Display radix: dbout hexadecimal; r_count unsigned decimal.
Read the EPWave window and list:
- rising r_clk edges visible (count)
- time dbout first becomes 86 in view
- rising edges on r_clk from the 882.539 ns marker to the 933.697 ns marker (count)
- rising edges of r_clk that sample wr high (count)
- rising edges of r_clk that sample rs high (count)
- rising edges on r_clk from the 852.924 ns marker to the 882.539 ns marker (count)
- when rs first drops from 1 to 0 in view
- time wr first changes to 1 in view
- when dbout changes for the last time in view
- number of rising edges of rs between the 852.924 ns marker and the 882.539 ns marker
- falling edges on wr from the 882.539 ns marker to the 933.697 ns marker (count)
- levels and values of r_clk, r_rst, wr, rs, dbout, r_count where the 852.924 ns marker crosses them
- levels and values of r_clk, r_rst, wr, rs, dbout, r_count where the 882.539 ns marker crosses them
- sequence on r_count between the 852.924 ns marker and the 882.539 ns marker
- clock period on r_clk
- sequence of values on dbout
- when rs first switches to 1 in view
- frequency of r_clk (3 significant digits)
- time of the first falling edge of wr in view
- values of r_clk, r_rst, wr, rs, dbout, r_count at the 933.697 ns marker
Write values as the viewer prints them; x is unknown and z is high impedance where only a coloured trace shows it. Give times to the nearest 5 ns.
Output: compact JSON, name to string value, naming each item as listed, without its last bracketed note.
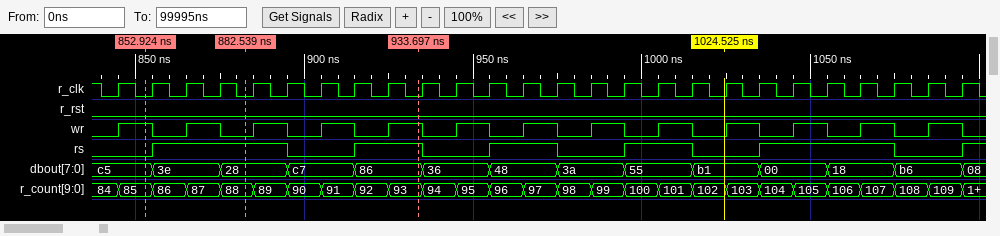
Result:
{"rising r_clk edges visible": "26", "time dbout first becomes 86 in view": "915 ns", "rising edges on r_clk from the 882.539 ns marker to the 933.697 ns marker": "5", "rising edges of r_clk that sample wr high": "13", "rising edges of r_clk that sample rs high": "14", "rising edges on r_clk from the 852.924 ns marker to the 882.539 ns marker": "3", "when rs first drops from 1 to 0 in view": "895 ns", "time wr first changes to 1 in view": "845 ns", "when dbout changes for the last time in view": "1095 ns", "number of rising edges of rs between the 852.924 ns marker and the 882.539 ns marker": "1", "falling edges on wr from the 882.539 ns marker to the 933.697 ns marker": "2", "levels and values of r_clk, r_rst, wr, rs, dbout, r_count where the 852.924 ns marker crosses them": "r_clk=0, r_rst=0, wr=1, rs=0, dbout=c5, r_count=85", "levels and values of r_clk, r_rst, wr, rs, dbout, r_count where the 882.539 ns marker crosses them": "r_clk=0, r_rst=0, wr=0, rs=1, dbout=28, r_count=88", "sequence on r_count between the 852.924 ns marker and the 882.539 ns marker": "85, 86, 87, 88", "clock period on r_clk": "10 ns", "sequence of values on dbout": "c5, 3e, 28, c7, 86, 36, 48, 3a, 55, b1, 00, 18, b6, 08", "when rs first switches to 1 in view": "855 ns", "frequency of r_clk": "100 MHz", "time of the first falling edge of wr in view": "855 ns", "values of r_clk, r_rst, wr, rs, dbout, r_count at the 933.697 ns marker": "r_clk=0, r_rst=0, wr=1, rs=1, dbout=86, r_count=93"}
